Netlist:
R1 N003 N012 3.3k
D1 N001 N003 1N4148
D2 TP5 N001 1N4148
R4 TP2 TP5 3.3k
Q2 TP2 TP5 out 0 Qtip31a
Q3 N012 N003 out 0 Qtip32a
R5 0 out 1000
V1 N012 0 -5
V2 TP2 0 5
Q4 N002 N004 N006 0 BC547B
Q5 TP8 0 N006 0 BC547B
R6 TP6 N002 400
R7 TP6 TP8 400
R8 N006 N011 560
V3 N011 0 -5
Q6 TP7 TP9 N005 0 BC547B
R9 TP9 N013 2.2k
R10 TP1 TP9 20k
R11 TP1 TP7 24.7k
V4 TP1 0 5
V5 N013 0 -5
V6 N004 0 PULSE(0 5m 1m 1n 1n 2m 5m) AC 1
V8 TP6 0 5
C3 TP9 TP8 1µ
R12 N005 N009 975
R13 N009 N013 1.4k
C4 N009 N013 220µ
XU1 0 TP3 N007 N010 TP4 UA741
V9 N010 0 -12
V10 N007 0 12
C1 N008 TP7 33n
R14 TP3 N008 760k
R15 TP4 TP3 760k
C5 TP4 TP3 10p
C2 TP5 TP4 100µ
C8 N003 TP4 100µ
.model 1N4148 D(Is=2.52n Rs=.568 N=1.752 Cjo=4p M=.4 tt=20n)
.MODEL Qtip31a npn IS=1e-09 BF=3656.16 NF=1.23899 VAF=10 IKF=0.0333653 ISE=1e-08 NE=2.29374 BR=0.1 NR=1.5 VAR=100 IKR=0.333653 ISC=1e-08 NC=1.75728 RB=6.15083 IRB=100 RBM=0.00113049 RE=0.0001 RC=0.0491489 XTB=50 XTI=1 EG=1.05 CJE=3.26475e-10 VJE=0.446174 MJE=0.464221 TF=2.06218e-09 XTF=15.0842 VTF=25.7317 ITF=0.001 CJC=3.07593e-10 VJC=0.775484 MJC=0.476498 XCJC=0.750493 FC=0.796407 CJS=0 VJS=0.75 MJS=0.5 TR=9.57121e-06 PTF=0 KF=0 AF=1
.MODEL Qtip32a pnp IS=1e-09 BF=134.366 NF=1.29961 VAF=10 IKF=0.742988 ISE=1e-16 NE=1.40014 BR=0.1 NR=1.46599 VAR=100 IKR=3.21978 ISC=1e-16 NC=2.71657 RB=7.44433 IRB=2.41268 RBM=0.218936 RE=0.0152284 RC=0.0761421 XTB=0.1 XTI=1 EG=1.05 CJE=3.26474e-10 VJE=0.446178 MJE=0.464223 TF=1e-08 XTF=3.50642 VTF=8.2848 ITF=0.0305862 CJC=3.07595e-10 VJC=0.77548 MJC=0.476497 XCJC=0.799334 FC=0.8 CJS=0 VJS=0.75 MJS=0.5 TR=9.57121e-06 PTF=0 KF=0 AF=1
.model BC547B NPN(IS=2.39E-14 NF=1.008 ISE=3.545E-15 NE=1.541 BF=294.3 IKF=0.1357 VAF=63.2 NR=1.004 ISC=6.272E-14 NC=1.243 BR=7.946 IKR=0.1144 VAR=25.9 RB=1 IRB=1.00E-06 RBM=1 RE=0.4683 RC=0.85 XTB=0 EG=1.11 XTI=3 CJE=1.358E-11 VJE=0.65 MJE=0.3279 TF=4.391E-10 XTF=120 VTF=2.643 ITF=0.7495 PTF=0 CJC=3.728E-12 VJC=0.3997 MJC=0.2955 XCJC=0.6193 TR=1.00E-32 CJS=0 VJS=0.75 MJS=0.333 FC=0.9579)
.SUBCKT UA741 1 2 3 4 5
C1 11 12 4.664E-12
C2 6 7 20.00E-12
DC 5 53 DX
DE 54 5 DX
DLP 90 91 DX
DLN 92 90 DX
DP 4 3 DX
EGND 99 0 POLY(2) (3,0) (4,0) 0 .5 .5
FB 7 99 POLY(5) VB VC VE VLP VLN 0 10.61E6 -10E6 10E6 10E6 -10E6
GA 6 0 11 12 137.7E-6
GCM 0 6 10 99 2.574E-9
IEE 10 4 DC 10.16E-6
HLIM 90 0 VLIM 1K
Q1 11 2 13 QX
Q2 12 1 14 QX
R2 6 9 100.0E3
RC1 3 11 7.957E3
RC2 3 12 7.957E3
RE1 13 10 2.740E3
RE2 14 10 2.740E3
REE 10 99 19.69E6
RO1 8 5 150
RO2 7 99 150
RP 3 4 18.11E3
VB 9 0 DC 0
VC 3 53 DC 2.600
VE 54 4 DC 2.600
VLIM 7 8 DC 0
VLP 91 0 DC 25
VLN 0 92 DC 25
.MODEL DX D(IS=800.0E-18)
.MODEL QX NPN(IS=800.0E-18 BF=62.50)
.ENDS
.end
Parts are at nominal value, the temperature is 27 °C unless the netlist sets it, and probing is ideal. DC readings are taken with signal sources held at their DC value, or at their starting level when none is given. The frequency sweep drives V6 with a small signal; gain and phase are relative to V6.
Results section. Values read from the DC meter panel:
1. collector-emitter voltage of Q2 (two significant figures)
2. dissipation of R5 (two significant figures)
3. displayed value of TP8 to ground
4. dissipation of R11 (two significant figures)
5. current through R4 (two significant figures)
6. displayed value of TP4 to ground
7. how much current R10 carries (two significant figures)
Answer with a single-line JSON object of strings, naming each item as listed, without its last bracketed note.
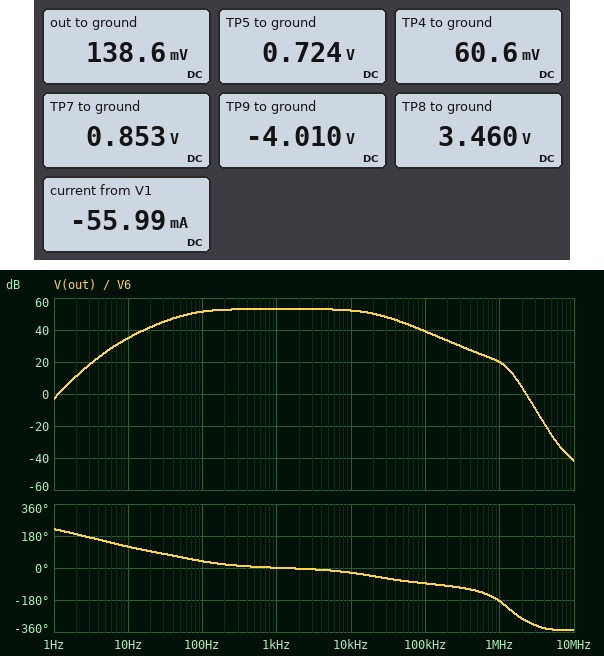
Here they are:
{"collector-emitter voltage of Q2": "4.9 V", "dissipation of R5": "19 µW", "displayed value of TP8 to ground": "3.460 V", "dissipation of R11": "700 µW", "current through R4": "1.3 mA", "displayed value of TP4 to ground": "60.6 mV", "how much current R10 carries": "450 µA"}
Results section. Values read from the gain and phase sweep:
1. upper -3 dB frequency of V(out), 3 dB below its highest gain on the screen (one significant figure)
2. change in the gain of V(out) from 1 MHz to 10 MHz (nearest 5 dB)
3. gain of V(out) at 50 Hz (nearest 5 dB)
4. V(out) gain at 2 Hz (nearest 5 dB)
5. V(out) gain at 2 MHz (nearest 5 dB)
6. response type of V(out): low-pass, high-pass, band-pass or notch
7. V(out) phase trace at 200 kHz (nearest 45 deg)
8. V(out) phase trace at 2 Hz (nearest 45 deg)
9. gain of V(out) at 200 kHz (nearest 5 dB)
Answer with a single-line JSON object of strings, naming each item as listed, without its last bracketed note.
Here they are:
{"upper -3 dB frequency of V(out), 3 dB below its highest gain on the screen": "20 kHz", "change in the gain of V(out) from 1 MHz to 10 MHz": "-60 dB", "gain of V(out) at 50 Hz": "50 dB", "V(out) gain at 2 Hz": "10 dB", "V(out) gain at 2 MHz": "5 dB", "response type of V(out): low-pass, high-pass, band-pass or notch": "band-pass", "V(out) phase trace at 200 kHz": "-90 deg", "V(out) phase trace at 2 Hz": "180 deg", "gain of V(out) at 200 kHz": "35 dB"}
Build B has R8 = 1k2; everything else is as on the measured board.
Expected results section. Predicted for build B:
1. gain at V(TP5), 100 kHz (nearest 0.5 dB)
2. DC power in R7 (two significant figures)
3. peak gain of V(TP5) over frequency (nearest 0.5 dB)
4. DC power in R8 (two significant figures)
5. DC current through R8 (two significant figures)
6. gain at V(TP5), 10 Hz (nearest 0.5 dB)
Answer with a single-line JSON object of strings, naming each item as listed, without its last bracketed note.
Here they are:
{"gain at V(TP5), 100 kHz": "33.0 dB", "DC power in R7": "1.3 mW", "peak gain of V(TP5) over frequency": "47.0 dB", "DC power in R8": "16 mW", "DC current through R8": "3.6 mA", "gain at V(TP5), 10 Hz": "29.0 dB"}
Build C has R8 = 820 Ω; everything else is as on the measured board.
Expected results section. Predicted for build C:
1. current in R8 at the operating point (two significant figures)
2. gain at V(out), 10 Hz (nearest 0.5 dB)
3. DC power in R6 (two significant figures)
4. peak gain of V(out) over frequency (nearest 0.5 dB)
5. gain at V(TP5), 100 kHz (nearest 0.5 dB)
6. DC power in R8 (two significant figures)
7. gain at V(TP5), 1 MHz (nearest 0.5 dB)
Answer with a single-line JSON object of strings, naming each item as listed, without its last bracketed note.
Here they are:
{"current in R8 at the operating point": "5.3 mA", "gain at V(out), 10 Hz": "32.0 dB", "DC power in R6": "2.8 mW", "peak gain of V(out) over frequency": "50.0 dB", "gain at V(TP5), 100 kHz": "36.0 dB", "DC power in R8": "23 mW", "gain at V(TP5), 1 MHz": "17.0 dB"}
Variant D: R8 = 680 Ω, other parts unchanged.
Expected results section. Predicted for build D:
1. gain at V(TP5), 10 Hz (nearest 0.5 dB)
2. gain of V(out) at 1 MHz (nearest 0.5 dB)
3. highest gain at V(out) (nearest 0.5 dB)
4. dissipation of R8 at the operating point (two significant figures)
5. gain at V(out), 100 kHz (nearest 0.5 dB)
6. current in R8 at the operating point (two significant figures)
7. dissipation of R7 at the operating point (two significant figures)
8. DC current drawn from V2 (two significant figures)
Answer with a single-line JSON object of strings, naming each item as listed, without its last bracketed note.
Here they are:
{"gain at V(TP5), 10 Hz": "33.5 dB", "gain of V(out) at 1 MHz": "18.5 dB", "highest gain at V(out)": "51.5 dB", "dissipation of R8 at the operating point": "28 mW", "gain at V(out), 100 kHz": "37.5 dB", "current in R8 at the operating point": "6.4 mA", "dissipation of R7 at the operating point": "4.0 mW", "DC current drawn from V2": "56 mA"}
